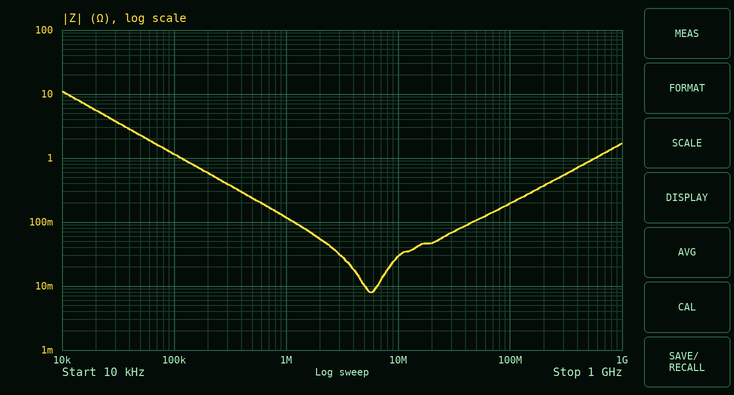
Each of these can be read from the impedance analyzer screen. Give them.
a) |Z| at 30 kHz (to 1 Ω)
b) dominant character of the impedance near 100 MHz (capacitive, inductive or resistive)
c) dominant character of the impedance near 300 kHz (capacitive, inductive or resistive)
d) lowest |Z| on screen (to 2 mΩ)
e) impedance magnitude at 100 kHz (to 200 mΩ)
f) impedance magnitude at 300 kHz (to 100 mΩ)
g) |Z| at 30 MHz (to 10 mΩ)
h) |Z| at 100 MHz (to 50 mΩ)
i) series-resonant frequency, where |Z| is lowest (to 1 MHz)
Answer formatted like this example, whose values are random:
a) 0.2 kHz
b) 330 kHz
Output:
a) 4 Ω
b) inductive
c) capacitive
d) 8 mΩ
e) 1.2 Ω
f) 400 mΩ
g) 70 mΩ
h) 200 mΩ
i) 6 MHz
